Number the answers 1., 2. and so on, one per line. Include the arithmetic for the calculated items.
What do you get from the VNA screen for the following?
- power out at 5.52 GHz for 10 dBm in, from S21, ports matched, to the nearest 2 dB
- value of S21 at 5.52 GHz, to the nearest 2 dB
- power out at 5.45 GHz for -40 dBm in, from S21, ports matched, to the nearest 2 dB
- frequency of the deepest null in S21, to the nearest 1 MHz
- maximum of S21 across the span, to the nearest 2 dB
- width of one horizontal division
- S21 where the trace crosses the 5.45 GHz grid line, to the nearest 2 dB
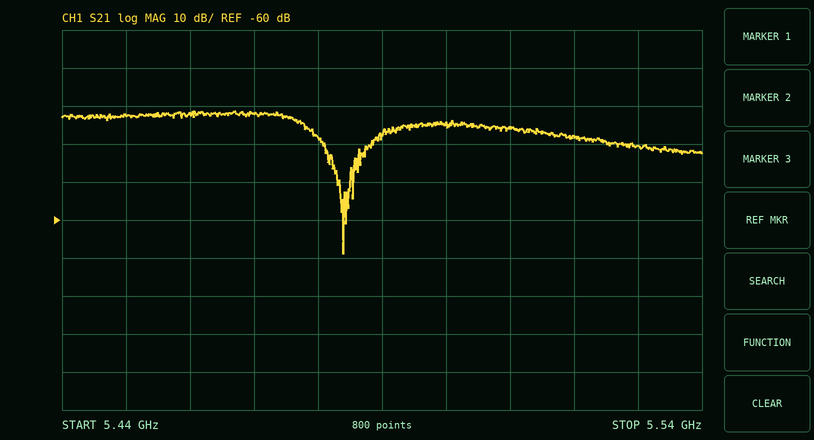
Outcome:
1. 10 dBm + (-38 dB) = -28 dBm
2. -38 dB
3. -40 dBm + (-32 dB) = -72 dBm
4. 5.484 GHz
5. -32 dB
6. 10 MHz
7. -32 dB
